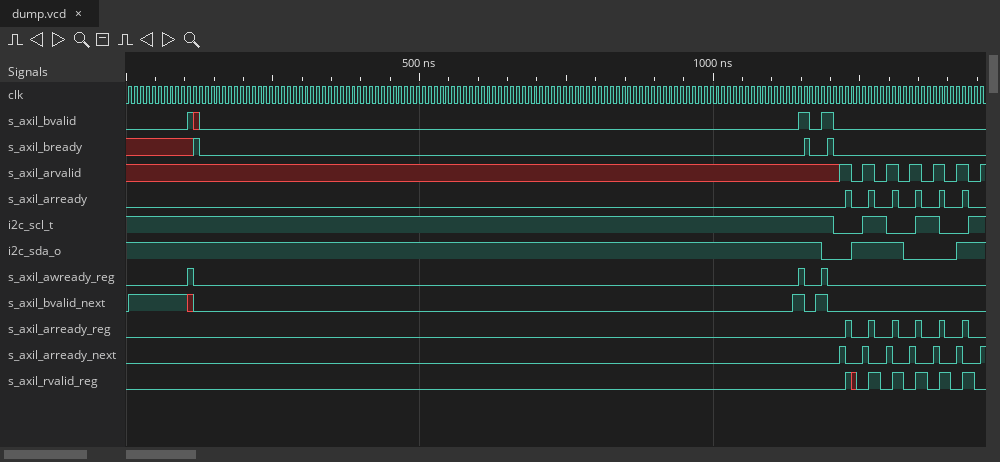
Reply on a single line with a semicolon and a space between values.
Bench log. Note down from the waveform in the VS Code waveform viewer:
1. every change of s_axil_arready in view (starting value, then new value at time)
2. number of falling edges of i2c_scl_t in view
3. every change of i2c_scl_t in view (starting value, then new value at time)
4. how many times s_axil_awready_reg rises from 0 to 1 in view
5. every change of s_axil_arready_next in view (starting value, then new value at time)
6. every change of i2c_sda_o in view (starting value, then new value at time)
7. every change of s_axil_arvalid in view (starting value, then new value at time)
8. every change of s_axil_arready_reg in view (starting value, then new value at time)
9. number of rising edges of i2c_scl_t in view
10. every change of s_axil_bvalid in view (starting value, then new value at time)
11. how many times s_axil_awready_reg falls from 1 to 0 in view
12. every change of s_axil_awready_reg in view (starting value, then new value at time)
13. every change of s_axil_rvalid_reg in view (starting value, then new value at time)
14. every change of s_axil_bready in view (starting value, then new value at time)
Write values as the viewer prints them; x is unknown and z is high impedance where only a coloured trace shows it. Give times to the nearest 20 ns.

0, 1 at 1220 ns, 0 at 1240 ns, 1 at 1260 ns, 0 at 1280 ns, 1 at 1300 ns, 0 at 1320 ns, 1 at 1340 ns, 0 at 1360 ns, 1 at 1380 ns, 0 at 1400 ns, 1 at 1420 ns, 0 at 1440 ns; 3; 1, 0 at 1200 ns, 1 at 1260 ns, 0 at 1300 ns, 1 at 1340 ns, 0 at 1380 ns, 1 at 1440 ns; 3; 0, 1 at 1220 ns, 0 at 1220 ns, 1 at 1260 ns, 0 at 1260 ns, 1 at 1300 ns, 0 at 1300 ns, 1 at 1340 ns, 0 at 1340 ns, 1 at 1380 ns, 0 at 1380 ns, 1 at 1420 ns, 0 at 1420 ns, 1 at 1460 ns; 1, 0 at 1180 ns, 1 at 1240 ns, 0 at 1320 ns, 1 at 1420 ns; x, 1 at 1220 ns, 0 at 1240 ns, 1 at 1260 ns, 0 at 1280 ns, 1 at 1300 ns, 0 at 1320 ns, 1 at 1340 ns, 0 at 1360 ns, 1 at 1380 ns, 0 at 1400 ns, 1 at 1420 ns, 0 at 1440 ns, 1 at 1460 ns; 0, 1 at 1220 ns, 0 at 1240 ns, 1 at 1260 ns, 0 at 1280 ns, 1 at 1300 ns, 0 at 1320 ns, 1 at 1340 ns, 0 at 1360 ns, 1 at 1380 ns, 0 at 1400 ns, 1 at 1420 ns, 0 at 1440 ns; 3; 0, 1 at 100 ns, x at 120 ns, 0 at 120 ns, 1 at 1140 ns, 0 at 1160 ns, 1 at 1180 ns, 0 at 1200 ns; 3; 0, 1 at 100 ns, 0 at 120 ns, 1 at 1140 ns, 0 at 1160 ns, 1 at 1180 ns, 0 at 1200 ns; 0, 1 at 1220 ns, x at 1240 ns, 0 at 1240 ns, 1 at 1260 ns, 0 at 1280 ns, 1 at 1300 ns, 0 at 1320 ns, 1 at 1340 ns, 0 at 1360 ns, 1 at 1380 ns, 0 at 1400 ns, 1 at 1420 ns, 0 at 1440 ns; x, 1 at 120 ns, 0 at 120 ns, 1 at 1160 ns, 0 at 1160 ns, 1 at 1200 ns, 0 at 1200 ns
